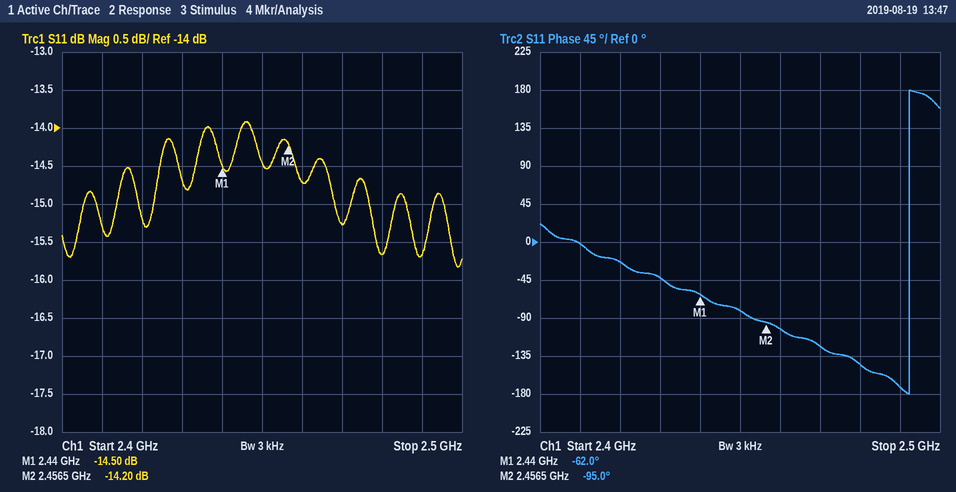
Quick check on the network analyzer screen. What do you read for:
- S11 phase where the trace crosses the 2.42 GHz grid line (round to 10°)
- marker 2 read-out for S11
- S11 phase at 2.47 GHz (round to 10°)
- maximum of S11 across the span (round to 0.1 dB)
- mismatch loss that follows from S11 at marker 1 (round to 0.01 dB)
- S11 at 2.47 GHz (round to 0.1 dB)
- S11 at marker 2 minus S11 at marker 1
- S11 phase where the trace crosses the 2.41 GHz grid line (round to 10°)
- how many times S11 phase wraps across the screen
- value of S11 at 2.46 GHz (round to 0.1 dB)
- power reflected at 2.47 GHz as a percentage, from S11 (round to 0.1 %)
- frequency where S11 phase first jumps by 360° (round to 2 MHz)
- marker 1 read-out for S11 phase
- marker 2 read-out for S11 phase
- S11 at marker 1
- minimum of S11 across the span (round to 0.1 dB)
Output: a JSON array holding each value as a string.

["-20°", "-14.20 dB", "-120°", "-13.9 dB", "0.16 dB", "-15.3 dB", "0.30 dB", "0°", "1", "-14.7 dB", "3.0 %", "2.492 GHz", "-62.0°", "-95.0°", "-14.50 dB", "-15.8 dB"]
